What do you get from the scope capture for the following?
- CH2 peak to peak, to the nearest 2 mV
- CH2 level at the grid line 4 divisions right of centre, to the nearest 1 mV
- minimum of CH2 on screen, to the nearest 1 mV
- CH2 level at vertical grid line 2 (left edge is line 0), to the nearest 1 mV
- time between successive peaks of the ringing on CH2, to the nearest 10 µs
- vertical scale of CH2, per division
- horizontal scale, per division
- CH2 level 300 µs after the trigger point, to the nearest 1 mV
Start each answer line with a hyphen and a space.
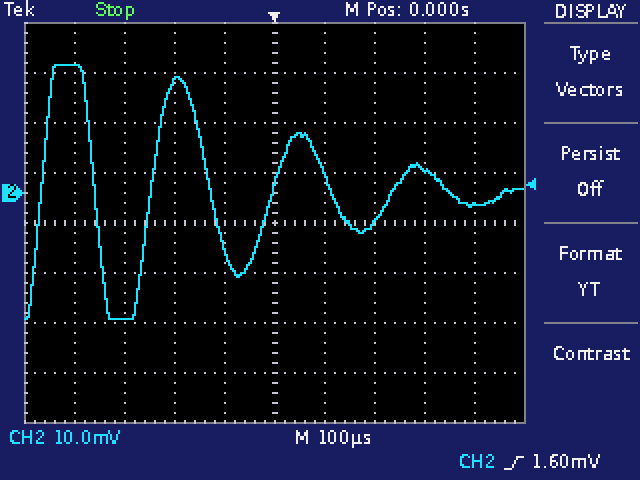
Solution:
- 50 mV
- -2 mV
- -25 mV
- -25 mV
- 230 µs
- 10 mV
- 100 µs
- 5 mV
